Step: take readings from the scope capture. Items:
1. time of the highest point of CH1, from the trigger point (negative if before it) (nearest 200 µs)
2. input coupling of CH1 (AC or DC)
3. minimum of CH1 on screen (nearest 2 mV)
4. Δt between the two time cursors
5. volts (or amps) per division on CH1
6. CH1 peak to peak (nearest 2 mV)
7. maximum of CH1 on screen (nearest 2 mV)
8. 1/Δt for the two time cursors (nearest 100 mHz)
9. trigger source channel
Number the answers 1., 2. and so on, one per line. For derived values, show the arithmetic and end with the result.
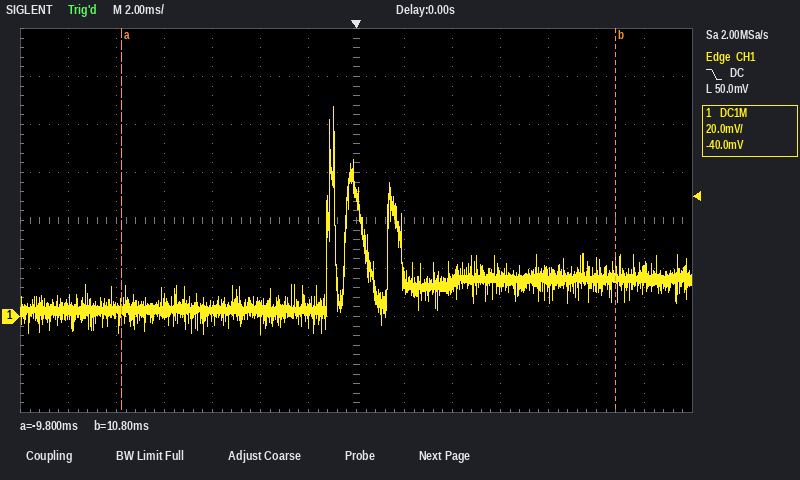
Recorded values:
1. -1.0 ms
2. DC
3. -8 mV
4. 10.8 ms − (-9.8 ms) = 20.6 ms
5. 20 mV
6. 88 mV − (-8 mV) = 96 mV
7. 88 mV
8. 1 / 20.6 ms ≈ 48.5 Hz
9. CH1
